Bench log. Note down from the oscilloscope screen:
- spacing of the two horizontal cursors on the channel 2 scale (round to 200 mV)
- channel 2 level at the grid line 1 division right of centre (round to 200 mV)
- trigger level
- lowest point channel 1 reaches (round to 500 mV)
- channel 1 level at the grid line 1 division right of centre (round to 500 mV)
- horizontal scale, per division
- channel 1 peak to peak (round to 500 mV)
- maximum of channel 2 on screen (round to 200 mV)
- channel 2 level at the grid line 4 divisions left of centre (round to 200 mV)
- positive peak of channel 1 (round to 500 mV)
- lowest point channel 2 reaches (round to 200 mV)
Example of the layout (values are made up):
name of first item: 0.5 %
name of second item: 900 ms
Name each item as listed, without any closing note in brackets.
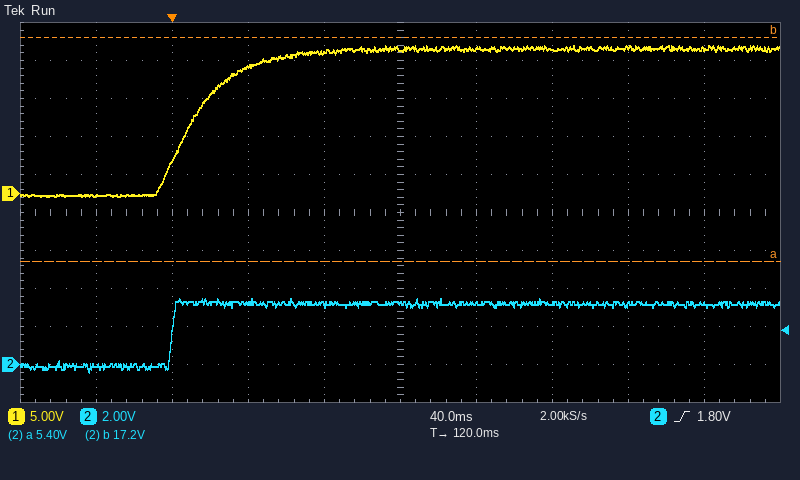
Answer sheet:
spacing of the two horizontal cursors on the channel 2 scale: 11.8 V
channel 2 level at the grid line 1 division right of centre: 3.2 V
trigger level: 1.80 V
lowest point channel 1 reaches: -500 mV
channel 1 level at the grid line 1 division right of centre: 19.0 V
horizontal scale, per division: 40 ms
channel 1 peak to peak: 20.0 V
maximum of channel 2 on screen: 3.4 V
channel 2 level at the grid line 4 divisions left of centre: -200 mV
positive peak of channel 1: 19.5 V
lowest point channel 2 reaches: -400 mV
